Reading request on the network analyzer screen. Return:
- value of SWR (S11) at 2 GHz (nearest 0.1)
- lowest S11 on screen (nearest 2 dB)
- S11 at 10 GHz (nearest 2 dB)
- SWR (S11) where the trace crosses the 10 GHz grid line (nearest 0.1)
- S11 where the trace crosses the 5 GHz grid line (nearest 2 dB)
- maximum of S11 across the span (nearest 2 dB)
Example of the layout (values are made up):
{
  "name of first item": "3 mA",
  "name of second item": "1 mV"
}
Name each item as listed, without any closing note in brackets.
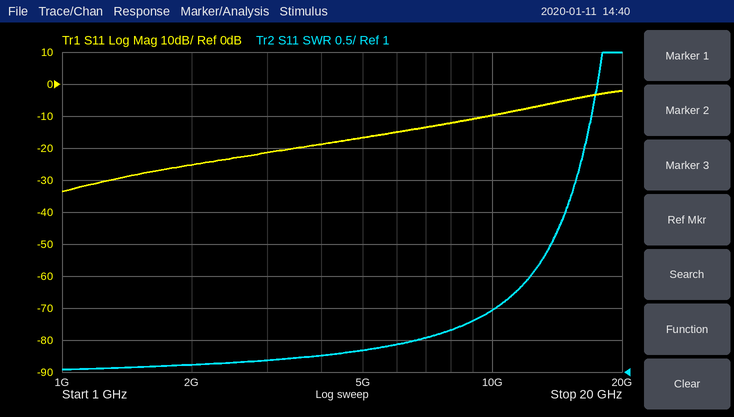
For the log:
{
  "value of SWR (S11) at 2 GHz": "1.1",
  "lowest S11 on screen": "-34 dB",
  "S11 at 10 GHz": "-10 dB",
  "SWR (S11) where the trace crosses the 10 GHz grid line": "2.0",
  "S11 where the trace crosses the 5 GHz grid line": "-16 dB",
  "maximum of S11 across the span": "-2 dB"
}
